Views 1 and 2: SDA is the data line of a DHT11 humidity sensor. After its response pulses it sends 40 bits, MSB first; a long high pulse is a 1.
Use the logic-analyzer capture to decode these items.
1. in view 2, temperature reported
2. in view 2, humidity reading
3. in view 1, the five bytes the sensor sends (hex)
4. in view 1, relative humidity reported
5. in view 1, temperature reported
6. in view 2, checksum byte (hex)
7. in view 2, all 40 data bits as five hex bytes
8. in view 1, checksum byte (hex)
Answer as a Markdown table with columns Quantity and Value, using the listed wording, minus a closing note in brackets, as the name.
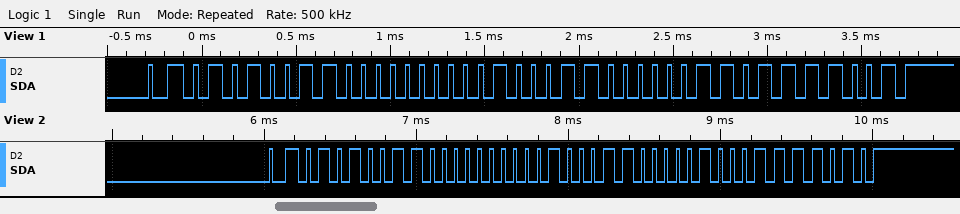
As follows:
| Quantity | Value |
|---|---|
| in view 2, temperature reported | 35.4 °C |
| in view 2, humidity reading | 83 % |
| in view 1, the five bytes the sensor sends | 53 00 23 03 79 |
| in view 1, relative humidity reported | 83 % |
| in view 1, temperature reported | 35.3 °C |
| in view 2, checksum byte | 0x7A |
| in view 2, all 40 data bits as five hex bytes | 53 00 23 04 7A |
| in view 1, checksum byte | 0x79 |
